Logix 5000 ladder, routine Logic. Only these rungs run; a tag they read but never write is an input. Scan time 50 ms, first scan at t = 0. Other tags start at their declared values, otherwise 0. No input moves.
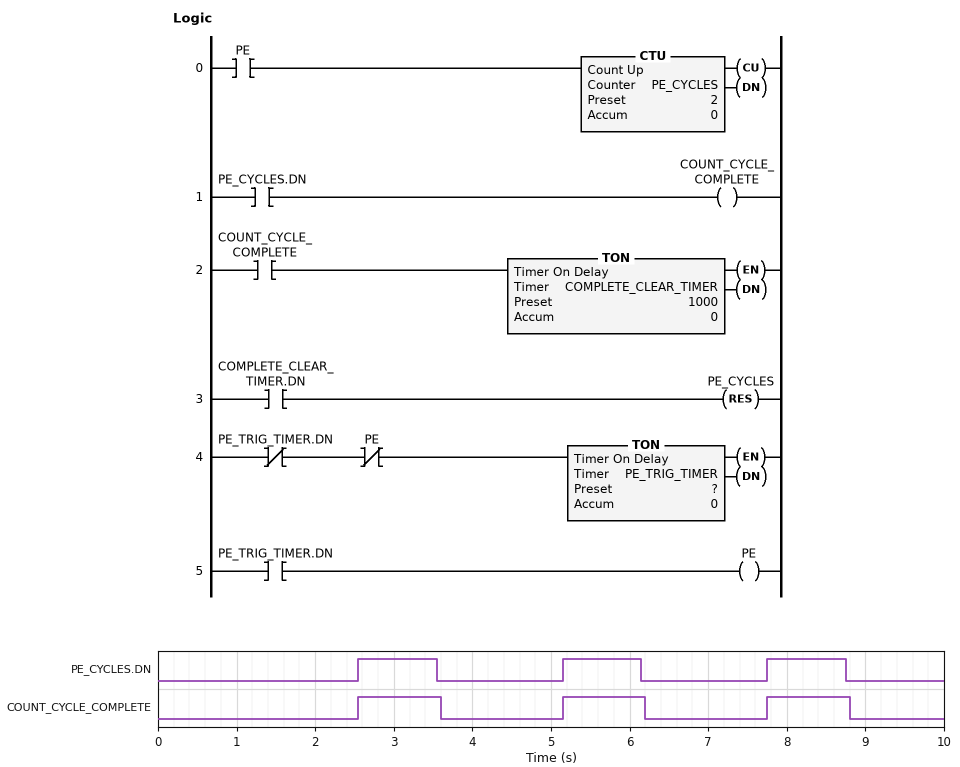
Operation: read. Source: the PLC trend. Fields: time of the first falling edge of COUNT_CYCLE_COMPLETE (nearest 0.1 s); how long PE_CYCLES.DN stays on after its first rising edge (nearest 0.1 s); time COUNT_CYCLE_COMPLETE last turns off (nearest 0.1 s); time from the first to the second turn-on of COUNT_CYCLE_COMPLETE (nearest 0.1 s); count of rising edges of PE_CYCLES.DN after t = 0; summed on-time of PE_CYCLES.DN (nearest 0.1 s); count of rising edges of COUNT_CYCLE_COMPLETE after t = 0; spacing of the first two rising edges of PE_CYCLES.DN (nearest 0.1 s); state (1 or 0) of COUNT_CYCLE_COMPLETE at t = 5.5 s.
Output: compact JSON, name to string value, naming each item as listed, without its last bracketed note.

{"time of the first falling edge of COUNT_CYCLE_COMPLETE": "3.6 s", "how long PE_CYCLES.DN stays on after its first rising edge": "1.0 s", "time COUNT_CYCLE_COMPLETE last turns off": "8.8 s", "time from the first to the second turn-on of COUNT_CYCLE_COMPLETE": "2.6 s", "count of rising edges of PE_CYCLES.DN after t = 0": "3", "summed on-time of PE_CYCLES.DN": "3.0 s", "count of rising edges of COUNT_CYCLE_COMPLETE after t = 0": "3", "spacing of the first two rising edges of PE_CYCLES.DN": "2.6 s", "state (1 or 0) of COUNT_CYCLE_COMPLETE at t = 5.5 s": "1"}
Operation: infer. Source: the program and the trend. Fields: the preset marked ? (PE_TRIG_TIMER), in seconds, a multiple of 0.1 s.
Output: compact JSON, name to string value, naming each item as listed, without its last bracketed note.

{"the preset marked ? (PE_TRIG_TIMER), in seconds, a multiple of 0.1 s": "1.2 s"}
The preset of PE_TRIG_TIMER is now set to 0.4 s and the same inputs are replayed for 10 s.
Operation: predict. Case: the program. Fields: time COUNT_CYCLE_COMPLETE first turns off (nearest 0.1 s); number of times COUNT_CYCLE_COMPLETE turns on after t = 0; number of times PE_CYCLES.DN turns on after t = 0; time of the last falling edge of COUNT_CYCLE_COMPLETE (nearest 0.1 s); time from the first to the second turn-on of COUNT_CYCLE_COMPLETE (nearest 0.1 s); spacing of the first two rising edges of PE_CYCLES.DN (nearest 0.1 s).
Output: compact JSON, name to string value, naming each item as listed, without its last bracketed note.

{"time COUNT_CYCLE_COMPLETE first turns off": "2.0 s", "number of times COUNT_CYCLE_COMPLETE turns on after t = 0": "5", "number of times PE_CYCLES.DN turns on after t = 0": "5", "time of the last falling edge of COUNT_CYCLE_COMPLETE": "8.0 s", "time from the first to the second turn-on of COUNT_CYCLE_COMPLETE": "2.0 s", "spacing of the first two rising edges of PE_CYCLES.DN": "2.0 s"}
